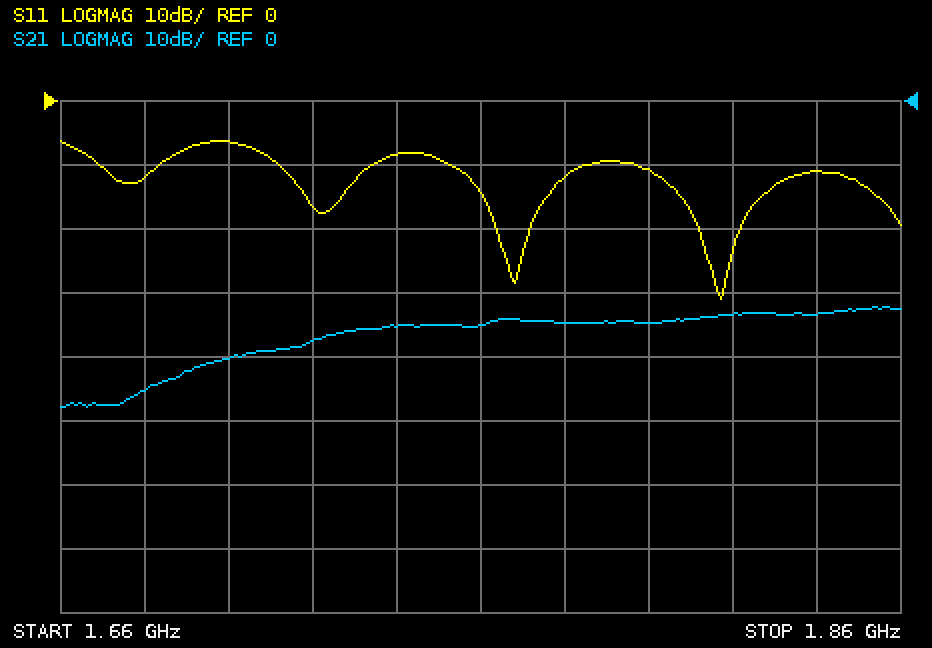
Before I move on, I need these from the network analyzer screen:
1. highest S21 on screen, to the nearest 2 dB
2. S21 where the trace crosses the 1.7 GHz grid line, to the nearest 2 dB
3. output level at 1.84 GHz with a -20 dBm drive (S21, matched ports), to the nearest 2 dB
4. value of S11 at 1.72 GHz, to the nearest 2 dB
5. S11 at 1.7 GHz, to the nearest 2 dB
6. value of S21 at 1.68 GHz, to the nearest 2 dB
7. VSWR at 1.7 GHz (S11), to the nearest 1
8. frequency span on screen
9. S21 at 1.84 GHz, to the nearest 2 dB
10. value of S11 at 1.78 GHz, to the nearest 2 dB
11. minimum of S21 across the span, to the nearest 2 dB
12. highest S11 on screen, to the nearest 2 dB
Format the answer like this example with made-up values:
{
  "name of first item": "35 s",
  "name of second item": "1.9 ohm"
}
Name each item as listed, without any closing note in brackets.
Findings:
{
  "highest S21 on screen, to the nearest 2 dB": "-32 dB",
  "S21 where the trace crosses the 1.7 GHz grid line, to the nearest 2 dB": "-40 dB",
  "output level at 1.84 GHz with a -20 dBm drive (S21, matched ports), to the nearest 2 dB": "-54 dBm",
  "value of S11 at 1.72 GHz, to the nearest 2 dB": "-16 dB",
  "S11 at 1.7 GHz, to the nearest 2 dB": "-6 dB",
  "value of S21 at 1.68 GHz, to the nearest 2 dB": "-46 dB",
  "VSWR at 1.7 GHz (S11), to the nearest 1": "3",
  "frequency span on screen": "200 MHz",
  "S21 at 1.84 GHz, to the nearest 2 dB": "-34 dB",
  "value of S11 at 1.78 GHz, to the nearest 2 dB": "-12 dB",
  "minimum of S21 across the span, to the nearest 2 dB": "-48 dB",
  "highest S11 on screen, to the nearest 2 dB": "-6 dB"
}
